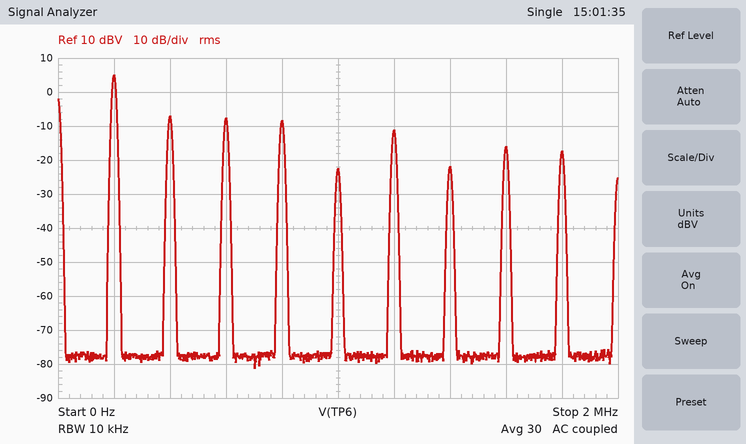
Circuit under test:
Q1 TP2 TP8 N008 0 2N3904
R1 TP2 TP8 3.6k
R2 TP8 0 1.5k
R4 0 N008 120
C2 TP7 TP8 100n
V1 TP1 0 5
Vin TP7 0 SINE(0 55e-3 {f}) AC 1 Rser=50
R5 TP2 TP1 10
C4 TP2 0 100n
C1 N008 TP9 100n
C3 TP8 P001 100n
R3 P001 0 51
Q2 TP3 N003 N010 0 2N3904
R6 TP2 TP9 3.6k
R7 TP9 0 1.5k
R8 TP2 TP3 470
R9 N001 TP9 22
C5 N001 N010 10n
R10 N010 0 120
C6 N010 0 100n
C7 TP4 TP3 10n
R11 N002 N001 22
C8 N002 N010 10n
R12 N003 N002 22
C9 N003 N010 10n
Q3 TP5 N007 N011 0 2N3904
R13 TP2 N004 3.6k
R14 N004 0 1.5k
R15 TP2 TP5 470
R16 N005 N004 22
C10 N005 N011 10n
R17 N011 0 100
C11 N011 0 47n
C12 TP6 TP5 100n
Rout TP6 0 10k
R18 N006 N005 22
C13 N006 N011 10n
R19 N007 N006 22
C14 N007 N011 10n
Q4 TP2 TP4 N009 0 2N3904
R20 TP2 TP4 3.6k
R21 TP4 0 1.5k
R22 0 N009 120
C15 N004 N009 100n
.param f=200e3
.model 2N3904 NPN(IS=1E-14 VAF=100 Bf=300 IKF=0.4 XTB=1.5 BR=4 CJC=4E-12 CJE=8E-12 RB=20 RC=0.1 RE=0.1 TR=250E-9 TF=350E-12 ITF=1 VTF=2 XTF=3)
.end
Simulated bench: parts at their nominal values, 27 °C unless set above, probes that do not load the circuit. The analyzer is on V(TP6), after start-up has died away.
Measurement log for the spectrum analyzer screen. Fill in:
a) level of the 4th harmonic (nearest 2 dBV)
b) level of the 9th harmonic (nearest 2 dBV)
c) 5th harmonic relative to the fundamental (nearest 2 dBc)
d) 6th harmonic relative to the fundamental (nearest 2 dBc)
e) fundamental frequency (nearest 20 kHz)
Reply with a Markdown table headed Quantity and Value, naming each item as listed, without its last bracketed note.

| Quantity | Value |
|---|---|
| level of the 4th harmonic | -8 dBV |
| level of the 9th harmonic | -18 dBV |
| 5th harmonic relative to the fundamental | -28 dBc |
| 6th harmonic relative to the fundamental | -16 dBc |
| fundamental frequency | 200 kHz |
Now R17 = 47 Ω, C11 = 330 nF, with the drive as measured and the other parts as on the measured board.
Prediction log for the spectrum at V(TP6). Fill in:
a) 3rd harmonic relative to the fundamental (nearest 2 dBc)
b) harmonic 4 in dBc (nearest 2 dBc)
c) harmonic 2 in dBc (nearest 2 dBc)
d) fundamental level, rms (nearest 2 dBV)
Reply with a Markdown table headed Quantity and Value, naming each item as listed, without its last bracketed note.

| Quantity | Value |
|---|---|
| 3rd harmonic relative to the fundamental | -10 dBc |
| harmonic 4 in dBc | -18 dBc |
| harmonic 2 in dBc | -18 dBc |
| fundamental level, rms | 6 dBV |
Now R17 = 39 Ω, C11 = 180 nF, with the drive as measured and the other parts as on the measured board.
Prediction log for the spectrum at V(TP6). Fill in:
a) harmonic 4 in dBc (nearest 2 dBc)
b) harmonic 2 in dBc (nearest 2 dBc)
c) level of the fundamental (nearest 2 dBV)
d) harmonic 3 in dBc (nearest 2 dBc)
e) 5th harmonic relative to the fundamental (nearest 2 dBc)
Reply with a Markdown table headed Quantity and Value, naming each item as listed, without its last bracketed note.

| Quantity | Value |
|---|---|
| harmonic 4 in dBc | -20 dBc |
| harmonic 2 in dBc | -20 dBc |
| level of the fundamental | 6 dBV |
| harmonic 3 in dBc | -10 dBc |
| 5th harmonic relative to the fundamental | -16 dBc |
